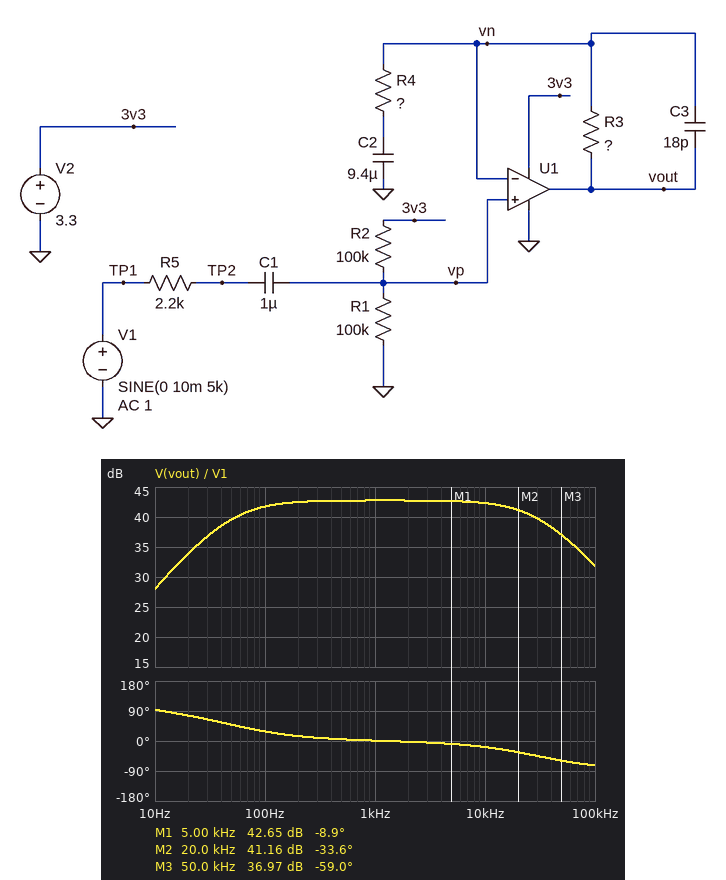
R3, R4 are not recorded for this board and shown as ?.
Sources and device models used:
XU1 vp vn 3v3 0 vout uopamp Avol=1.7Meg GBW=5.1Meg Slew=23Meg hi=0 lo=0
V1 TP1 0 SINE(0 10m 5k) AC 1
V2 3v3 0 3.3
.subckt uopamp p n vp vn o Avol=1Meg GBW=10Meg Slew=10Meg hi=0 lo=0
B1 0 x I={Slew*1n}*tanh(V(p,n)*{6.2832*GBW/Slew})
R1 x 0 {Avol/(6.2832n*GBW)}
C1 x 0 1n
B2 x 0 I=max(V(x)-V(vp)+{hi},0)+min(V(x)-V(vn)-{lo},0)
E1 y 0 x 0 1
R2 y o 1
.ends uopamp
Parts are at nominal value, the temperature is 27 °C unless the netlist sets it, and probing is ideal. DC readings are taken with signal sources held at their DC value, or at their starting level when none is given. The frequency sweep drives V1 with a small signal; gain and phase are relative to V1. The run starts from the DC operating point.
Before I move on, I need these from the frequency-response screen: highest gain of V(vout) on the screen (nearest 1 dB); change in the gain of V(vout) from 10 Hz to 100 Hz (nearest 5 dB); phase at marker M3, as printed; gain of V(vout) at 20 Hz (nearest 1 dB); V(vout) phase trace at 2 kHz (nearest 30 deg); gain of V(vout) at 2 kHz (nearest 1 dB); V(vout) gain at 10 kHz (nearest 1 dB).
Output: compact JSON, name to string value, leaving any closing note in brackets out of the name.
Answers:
{"highest gain of V(vout) on the screen": "43 dB", "change in the gain of V(vout) from 10 Hz to 100 Hz": "15 dB", "phase at marker M3, as printed": "-59.0 deg", "gain of V(vout) at 20 Hz": "34 dB", "V(vout) phase trace at 2 kHz": "0 deg", "gain of V(vout) at 2 kHz": "43 dB", "V(vout) gain at 10 kHz": "42 dB"}
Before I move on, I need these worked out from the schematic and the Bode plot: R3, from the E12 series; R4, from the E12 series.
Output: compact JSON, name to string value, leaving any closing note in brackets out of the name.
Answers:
{"R3, from the E12 series": "47 kΩ", "R4, from the E12 series": "330 Ω"}
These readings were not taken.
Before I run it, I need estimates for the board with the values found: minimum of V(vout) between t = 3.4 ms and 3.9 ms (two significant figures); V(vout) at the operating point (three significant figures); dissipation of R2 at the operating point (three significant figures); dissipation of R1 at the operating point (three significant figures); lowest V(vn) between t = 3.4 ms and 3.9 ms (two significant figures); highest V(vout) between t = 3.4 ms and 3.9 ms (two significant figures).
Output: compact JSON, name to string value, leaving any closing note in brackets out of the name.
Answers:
{"minimum of V(vout) between t = 3.4 ms and 3.9 ms": "290 mV", "V(vout) at the operating point": "1.65 V", "dissipation of R2 at the operating point": "27.2 µW", "dissipation of R1 at the operating point": "27.2 µW", "lowest V(vn) between t = 3.4 ms and 3.9 ms": "1.6 V", "highest V(vout) between t = 3.4 ms and 3.9 ms": "3.0 V"}
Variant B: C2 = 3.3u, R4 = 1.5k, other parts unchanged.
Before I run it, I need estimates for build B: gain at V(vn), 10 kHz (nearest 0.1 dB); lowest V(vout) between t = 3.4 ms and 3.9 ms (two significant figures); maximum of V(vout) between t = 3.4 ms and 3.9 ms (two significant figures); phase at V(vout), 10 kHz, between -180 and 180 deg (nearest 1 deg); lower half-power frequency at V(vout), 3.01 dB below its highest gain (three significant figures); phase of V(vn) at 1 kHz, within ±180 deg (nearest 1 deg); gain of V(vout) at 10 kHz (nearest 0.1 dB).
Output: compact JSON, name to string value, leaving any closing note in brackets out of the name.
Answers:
{"gain at V(vn), 10 kHz": "-0.4 dB", "lowest V(vout) between t = 3.4 ms and 3.9 ms": "1.3 V", "maximum of V(vout) between t = 3.4 ms and 3.9 ms": "2.0 V", "phase at V(vout), 10 kHz, between -180 and 180 deg": "-6 deg", "lower half-power frequency at V(vout), 3.01 dB below its highest gain": "32.4 Hz", "phase of V(vn) at 1 kHz, within ±180 deg": "0 deg", "gain of V(vout) at 10 kHz": "29.8 dB"}
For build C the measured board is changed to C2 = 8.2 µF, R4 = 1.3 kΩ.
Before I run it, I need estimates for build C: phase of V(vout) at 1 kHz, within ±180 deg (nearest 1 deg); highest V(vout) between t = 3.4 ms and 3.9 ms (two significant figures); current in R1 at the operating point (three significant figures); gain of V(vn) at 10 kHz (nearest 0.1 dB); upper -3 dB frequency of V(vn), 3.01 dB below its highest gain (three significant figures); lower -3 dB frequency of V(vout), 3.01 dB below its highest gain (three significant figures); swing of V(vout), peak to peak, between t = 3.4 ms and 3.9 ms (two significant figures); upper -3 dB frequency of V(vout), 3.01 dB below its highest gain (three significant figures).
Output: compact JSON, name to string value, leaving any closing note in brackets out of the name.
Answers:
{"phase of V(vout) at 1 kHz, within ±180 deg": "0 deg", "highest V(vout) between t = 3.4 ms and 3.9 ms": "2.0 V", "current in R1 at the operating point": "16.5 µA", "gain of V(vn) at 10 kHz": "-0.4 dB", "upper -3 dB frequency of V(vn), 3.01 dB below its highest gain": "99.9 kHz", "lower -3 dB frequency of V(vout), 3.01 dB below its highest gain": "15.5 Hz", "swing of V(vout), peak to peak, between t = 3.4 ms and 3.9 ms": "710 mV", "upper -3 dB frequency of V(vout), 3.01 dB below its highest gain": "79.9 kHz"}
